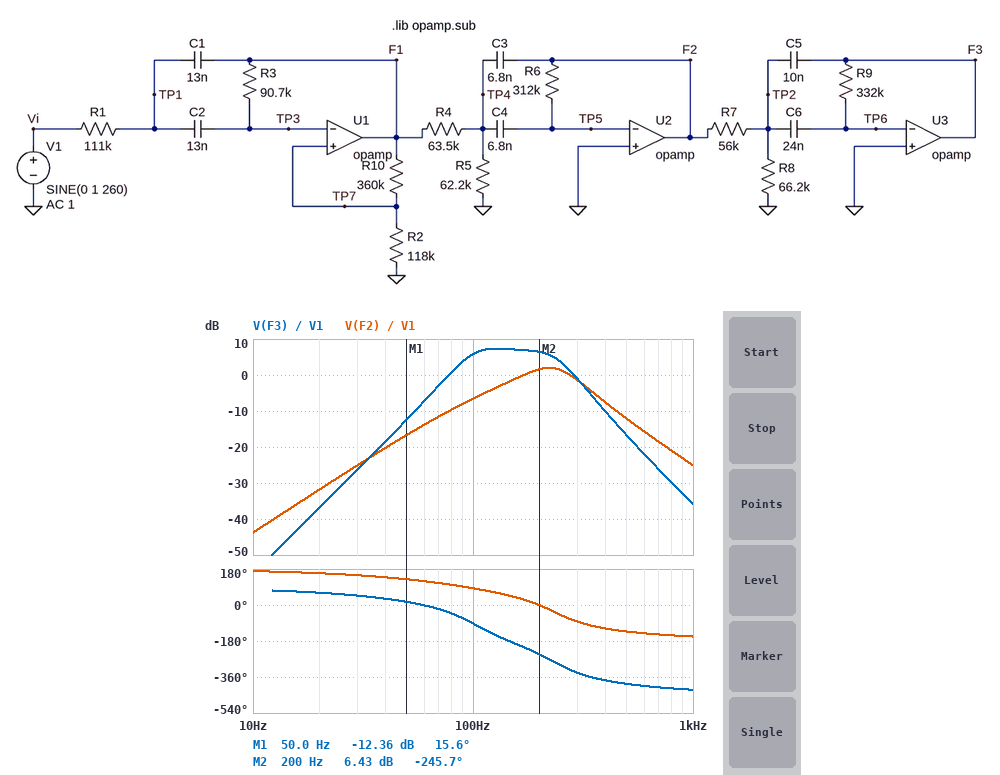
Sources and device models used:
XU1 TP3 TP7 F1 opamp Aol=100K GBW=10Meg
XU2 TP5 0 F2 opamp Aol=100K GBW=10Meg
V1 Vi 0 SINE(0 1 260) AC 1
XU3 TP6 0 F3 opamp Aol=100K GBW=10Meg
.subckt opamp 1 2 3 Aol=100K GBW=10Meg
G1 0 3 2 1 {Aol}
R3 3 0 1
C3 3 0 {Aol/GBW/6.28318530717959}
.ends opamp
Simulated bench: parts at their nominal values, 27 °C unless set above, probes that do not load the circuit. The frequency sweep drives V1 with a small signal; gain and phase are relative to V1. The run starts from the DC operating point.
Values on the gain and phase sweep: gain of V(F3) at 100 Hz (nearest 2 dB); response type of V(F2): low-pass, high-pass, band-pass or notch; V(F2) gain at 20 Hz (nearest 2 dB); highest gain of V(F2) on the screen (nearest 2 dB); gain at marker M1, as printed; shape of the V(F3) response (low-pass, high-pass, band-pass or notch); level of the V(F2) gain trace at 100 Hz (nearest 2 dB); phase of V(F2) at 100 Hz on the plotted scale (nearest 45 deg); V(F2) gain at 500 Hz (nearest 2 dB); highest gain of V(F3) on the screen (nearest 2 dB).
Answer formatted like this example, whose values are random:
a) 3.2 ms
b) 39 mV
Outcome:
a) 6 dB
b) band-pass
c) -32 dB
d) 2 dB
e) -12.36 dB
f) band-pass
g) -6 dB
h) 90 deg
i) -12 dB
j) 8 dB
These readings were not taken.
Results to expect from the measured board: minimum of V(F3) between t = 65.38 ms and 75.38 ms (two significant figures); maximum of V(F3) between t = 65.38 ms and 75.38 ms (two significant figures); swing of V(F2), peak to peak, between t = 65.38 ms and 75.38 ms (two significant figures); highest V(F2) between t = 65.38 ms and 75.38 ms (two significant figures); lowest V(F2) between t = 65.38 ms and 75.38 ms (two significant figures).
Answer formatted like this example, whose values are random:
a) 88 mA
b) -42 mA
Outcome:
a) -1.4 V
b) 1.4 V
c) 2.2 V
d) 1.1 V
e) -1.1 V
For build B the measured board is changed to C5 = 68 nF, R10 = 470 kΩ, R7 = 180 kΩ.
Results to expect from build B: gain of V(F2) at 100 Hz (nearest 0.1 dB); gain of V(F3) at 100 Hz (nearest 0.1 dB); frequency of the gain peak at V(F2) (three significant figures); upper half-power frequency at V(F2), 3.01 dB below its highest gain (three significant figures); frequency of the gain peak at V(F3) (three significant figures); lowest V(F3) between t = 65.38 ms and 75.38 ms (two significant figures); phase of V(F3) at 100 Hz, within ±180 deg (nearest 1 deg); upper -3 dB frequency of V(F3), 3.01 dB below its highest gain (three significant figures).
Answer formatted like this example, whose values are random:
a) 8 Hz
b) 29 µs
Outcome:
a) -7.4 dB
b) -24.6 dB
c) 223 Hz
d) 293 Hz
e) 193 Hz
f) -52 mV
g) -170 deg
h) 261 Hz
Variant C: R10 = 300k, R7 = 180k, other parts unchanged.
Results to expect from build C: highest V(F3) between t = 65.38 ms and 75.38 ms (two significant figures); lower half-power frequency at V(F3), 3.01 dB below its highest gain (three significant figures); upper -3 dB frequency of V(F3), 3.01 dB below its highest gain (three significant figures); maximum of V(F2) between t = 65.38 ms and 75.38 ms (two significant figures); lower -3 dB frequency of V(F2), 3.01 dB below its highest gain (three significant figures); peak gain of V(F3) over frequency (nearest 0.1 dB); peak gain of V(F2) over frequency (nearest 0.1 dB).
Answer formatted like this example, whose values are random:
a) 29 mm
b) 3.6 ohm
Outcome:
a) 430 mV
b) 79.2 Hz
c) 254 Hz
d) 1.2 V
e) 155 Hz
f) -3.8 dB
g) 2.6 dB
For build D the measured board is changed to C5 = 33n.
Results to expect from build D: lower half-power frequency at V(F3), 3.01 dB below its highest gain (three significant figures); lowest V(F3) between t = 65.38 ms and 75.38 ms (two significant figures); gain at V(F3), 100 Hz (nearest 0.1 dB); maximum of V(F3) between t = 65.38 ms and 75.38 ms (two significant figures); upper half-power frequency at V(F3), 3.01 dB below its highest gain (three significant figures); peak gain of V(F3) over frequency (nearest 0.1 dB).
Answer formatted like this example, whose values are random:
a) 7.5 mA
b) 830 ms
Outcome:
a) 52.7 Hz
b) -380 mV
c) -5.6 dB
d) 380 mV
e) 257 Hz
f) -5.1 dB
